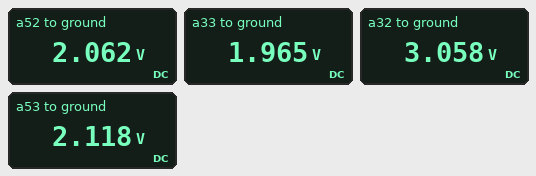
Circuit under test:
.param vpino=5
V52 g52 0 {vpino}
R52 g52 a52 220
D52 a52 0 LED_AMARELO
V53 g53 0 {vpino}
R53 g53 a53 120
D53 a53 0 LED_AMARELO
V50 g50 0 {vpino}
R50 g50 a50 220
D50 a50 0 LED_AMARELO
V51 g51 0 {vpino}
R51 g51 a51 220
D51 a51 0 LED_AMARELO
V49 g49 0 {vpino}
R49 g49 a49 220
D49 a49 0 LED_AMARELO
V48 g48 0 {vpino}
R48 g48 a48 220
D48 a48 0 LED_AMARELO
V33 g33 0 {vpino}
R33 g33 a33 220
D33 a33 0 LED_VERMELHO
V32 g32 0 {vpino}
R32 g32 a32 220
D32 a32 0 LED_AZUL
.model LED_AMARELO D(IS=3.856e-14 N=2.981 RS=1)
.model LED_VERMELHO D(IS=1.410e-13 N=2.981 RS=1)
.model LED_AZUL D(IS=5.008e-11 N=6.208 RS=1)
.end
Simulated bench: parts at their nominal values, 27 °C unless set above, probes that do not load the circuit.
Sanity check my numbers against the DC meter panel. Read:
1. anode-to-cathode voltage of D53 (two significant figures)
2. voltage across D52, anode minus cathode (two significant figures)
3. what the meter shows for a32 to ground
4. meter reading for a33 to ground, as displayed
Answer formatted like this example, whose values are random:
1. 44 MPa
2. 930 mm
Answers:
1. 2.1 V
2. 2.1 V
3. 3.058 V
4. 1.965 V
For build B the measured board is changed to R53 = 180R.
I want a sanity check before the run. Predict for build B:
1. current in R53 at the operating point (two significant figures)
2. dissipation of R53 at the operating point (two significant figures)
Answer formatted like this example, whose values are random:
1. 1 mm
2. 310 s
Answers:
1. 16 mA
2. 47 mW
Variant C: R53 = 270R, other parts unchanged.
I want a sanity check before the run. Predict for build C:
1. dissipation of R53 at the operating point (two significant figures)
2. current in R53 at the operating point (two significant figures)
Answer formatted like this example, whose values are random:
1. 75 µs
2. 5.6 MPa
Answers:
1. 32 mW
2. 11 mA
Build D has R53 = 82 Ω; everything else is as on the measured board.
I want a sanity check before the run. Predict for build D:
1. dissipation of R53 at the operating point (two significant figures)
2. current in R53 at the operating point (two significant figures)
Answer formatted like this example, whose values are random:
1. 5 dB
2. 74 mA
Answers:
1. 99 mW
2. 35 mA
